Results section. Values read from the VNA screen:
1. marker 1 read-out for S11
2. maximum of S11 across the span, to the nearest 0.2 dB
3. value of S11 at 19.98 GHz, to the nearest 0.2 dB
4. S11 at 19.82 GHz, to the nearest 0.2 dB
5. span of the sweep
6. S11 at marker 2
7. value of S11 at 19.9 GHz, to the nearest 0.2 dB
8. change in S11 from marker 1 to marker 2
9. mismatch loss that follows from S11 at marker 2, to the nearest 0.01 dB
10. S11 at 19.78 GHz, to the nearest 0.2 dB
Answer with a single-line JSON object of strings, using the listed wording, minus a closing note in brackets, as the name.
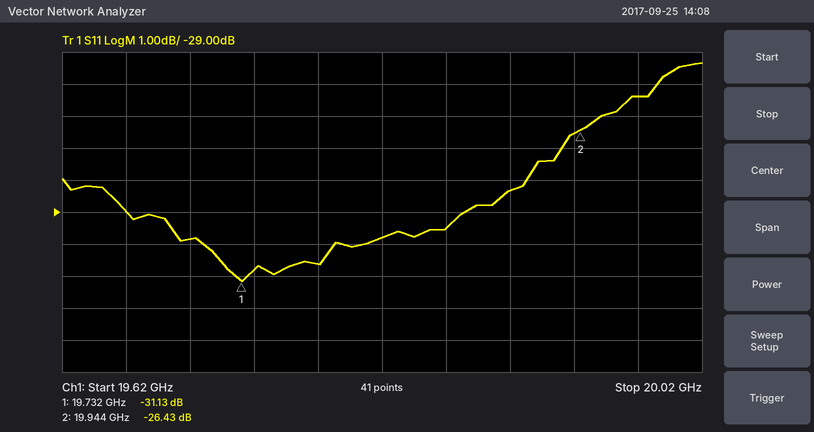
{"marker 1 read-out for S11": "-31.13 dB", "maximum of S11 across the span, to the nearest 0.2 dB": "-24.4 dB", "value of S11 at 19.98 GHz, to the nearest 0.2 dB": "-25.4 dB", "S11 at 19.82 GHz, to the nearest 0.2 dB": "-29.8 dB", "span of the sweep": "400 MHz", "S11 at marker 2": "-26.43 dB", "value of S11 at 19.9 GHz, to the nearest 0.2 dB": "-28.4 dB", "change in S11 from marker 1 to marker 2": "4.70 dB", "mismatch loss that follows from S11 at marker 2, to the nearest 0.01 dB": "0.01 dB", "S11 at 19.78 GHz, to the nearest 0.2 dB": "-30.6 dB"}
